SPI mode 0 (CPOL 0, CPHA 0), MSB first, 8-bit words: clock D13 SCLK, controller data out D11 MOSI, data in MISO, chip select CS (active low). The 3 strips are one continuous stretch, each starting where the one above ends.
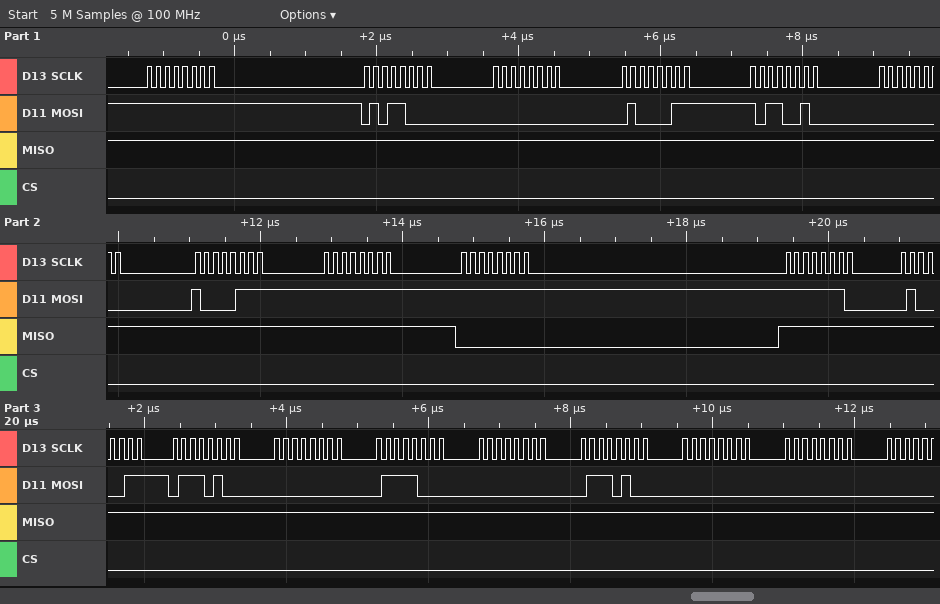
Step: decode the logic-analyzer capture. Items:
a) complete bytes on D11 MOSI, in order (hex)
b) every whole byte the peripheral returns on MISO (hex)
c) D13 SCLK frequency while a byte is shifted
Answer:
0xFF 0x58 0x00 0x43 0xB2 0x00 0x87 0xFF 0xFF 0xFE 0x43 0x74 0x00 0x78 0x00 0x74 0x00 0x00
0xFF 0xFF 0xFF 0xFF 0xFF 0xFF 0xFF 0xFF 0x00 0xFF 0xFF 0xFF 0xFF 0xFF 0xFF 0xFF 0xFF 0xFF
8 MHz
